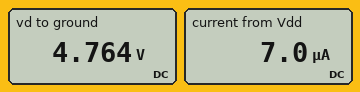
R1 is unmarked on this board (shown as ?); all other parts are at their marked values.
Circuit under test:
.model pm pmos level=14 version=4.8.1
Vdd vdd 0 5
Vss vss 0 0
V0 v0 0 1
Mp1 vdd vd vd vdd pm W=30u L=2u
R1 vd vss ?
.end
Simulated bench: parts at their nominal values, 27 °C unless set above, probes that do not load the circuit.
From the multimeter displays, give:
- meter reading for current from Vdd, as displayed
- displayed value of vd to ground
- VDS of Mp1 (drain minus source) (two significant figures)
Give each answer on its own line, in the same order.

7.0 µA
4.764 V
240 mV
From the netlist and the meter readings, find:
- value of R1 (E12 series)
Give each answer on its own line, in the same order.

680 kΩ
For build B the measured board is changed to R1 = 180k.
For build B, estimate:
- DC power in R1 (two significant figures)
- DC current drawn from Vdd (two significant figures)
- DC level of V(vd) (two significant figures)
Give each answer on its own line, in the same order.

120 µW
26 µA
4.7 V
